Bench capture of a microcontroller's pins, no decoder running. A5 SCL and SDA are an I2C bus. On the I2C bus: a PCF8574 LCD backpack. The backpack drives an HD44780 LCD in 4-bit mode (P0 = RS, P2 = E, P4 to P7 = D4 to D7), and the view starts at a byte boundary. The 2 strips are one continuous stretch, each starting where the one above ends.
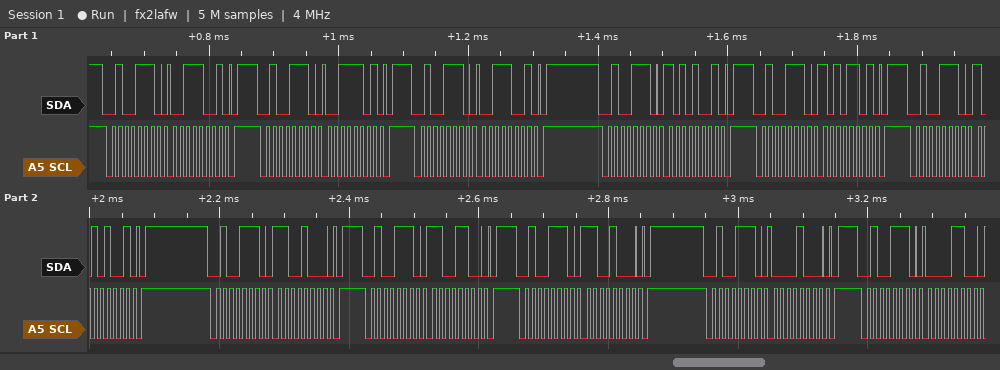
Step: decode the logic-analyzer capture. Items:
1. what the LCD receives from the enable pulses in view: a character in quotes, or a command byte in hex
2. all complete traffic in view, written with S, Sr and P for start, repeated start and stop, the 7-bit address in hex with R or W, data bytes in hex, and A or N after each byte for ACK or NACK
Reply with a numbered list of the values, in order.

1. ':'
2. S 27W A 39 A P S 27W A 3D A P S 27W A 39 A P S 27W A A9 A P S 27W A AD A P S 27W A A9 A P S 27W A C8 A P S 27W A CC A P S 27W A C8 A P S 27W A 08 A P S 27W A 0C A
